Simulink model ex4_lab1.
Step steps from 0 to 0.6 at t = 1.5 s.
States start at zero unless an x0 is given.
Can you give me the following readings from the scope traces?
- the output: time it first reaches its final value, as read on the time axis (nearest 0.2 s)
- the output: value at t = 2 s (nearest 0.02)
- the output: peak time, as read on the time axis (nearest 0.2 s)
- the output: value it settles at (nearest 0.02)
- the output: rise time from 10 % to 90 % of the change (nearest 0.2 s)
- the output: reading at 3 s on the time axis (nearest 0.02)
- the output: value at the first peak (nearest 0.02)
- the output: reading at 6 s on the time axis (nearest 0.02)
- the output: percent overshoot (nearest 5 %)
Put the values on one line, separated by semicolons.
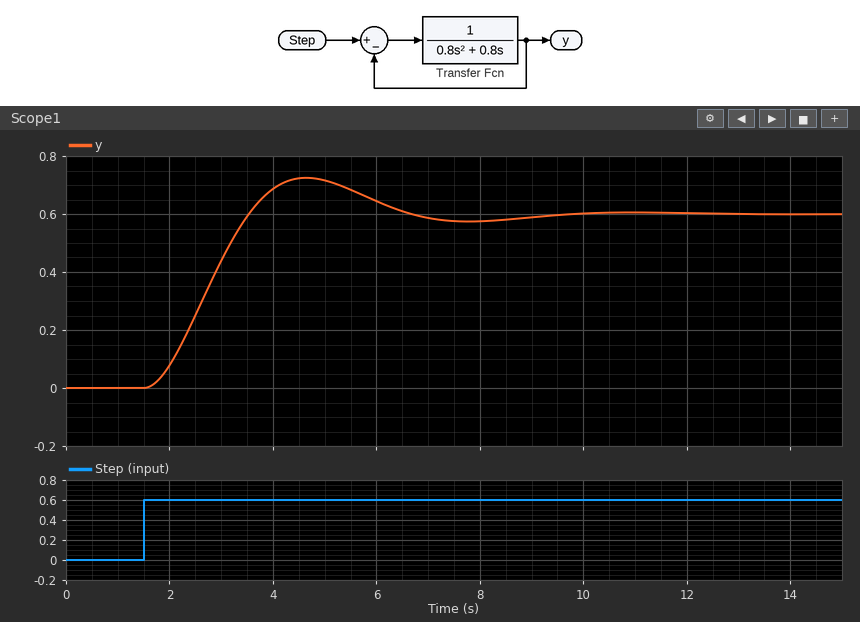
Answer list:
3.6 s; 0.08; 4.6 s; 0.60; 1.4 s; 0.44; 0.72; 0.64; 20 %
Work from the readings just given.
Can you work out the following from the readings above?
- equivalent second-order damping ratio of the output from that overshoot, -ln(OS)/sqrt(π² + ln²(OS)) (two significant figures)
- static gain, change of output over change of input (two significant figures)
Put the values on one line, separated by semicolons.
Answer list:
0.46; 1.0
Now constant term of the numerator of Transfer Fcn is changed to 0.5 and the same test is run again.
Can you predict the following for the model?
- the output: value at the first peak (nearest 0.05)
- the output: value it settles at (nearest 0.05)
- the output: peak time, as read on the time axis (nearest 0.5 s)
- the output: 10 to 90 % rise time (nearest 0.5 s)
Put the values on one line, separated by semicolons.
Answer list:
0.65; 0.60; 6.5 s; 2.5 s
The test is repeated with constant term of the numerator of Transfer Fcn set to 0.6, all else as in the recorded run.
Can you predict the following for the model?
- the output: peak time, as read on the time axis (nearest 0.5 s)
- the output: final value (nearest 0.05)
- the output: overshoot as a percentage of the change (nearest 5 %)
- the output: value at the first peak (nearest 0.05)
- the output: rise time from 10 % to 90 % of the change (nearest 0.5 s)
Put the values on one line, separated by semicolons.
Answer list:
6.0 s; 0.60; 10 %; 0.65; 2.0 s
